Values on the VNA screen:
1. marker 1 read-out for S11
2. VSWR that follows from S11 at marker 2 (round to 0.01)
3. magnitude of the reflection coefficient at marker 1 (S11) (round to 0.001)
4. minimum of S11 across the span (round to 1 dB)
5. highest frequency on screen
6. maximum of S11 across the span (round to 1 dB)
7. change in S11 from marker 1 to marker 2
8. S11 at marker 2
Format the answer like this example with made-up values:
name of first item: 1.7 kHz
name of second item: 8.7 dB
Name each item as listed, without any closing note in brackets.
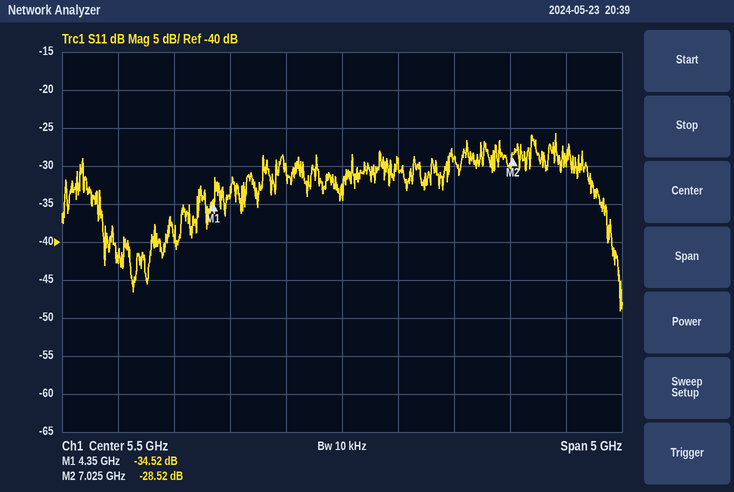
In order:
marker 1 read-out for S11: -34.52 dB
VSWR that follows from S11 at marker 2: 1.08
magnitude of the reflection coefficient at marker 1 (S11): 0.019
minimum of S11 across the span: -49 dB
highest frequency on screen: 8 GHz
maximum of S11 across the span: -26 dB
change in S11 from marker 1 to marker 2: 6.00 dB
S11 at marker 2: -28.52 dB
